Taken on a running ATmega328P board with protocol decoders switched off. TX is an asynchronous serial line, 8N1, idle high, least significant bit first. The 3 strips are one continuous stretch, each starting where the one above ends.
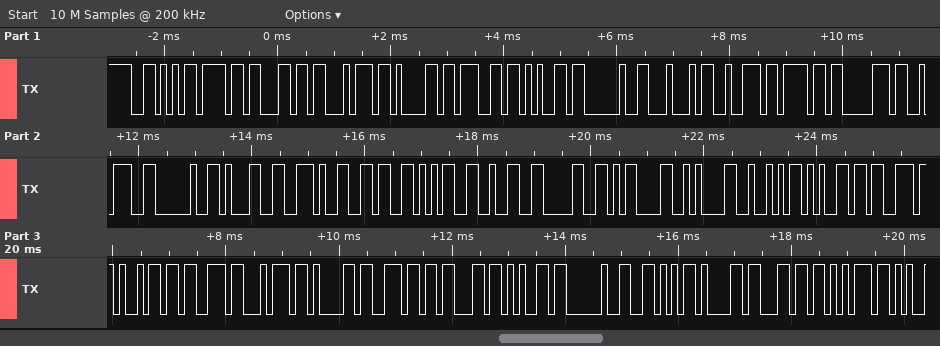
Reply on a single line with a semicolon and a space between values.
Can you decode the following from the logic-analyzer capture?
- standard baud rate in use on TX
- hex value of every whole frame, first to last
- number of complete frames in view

9600 baud; 56 6F 6C 74 61 67 65 20 44 72 6F 70 3A 20 31 2E 36 35 32 30 0D 0A 52 65 73 69 73 74 61 6E 63 65 20 56 61 6C 75; 37
